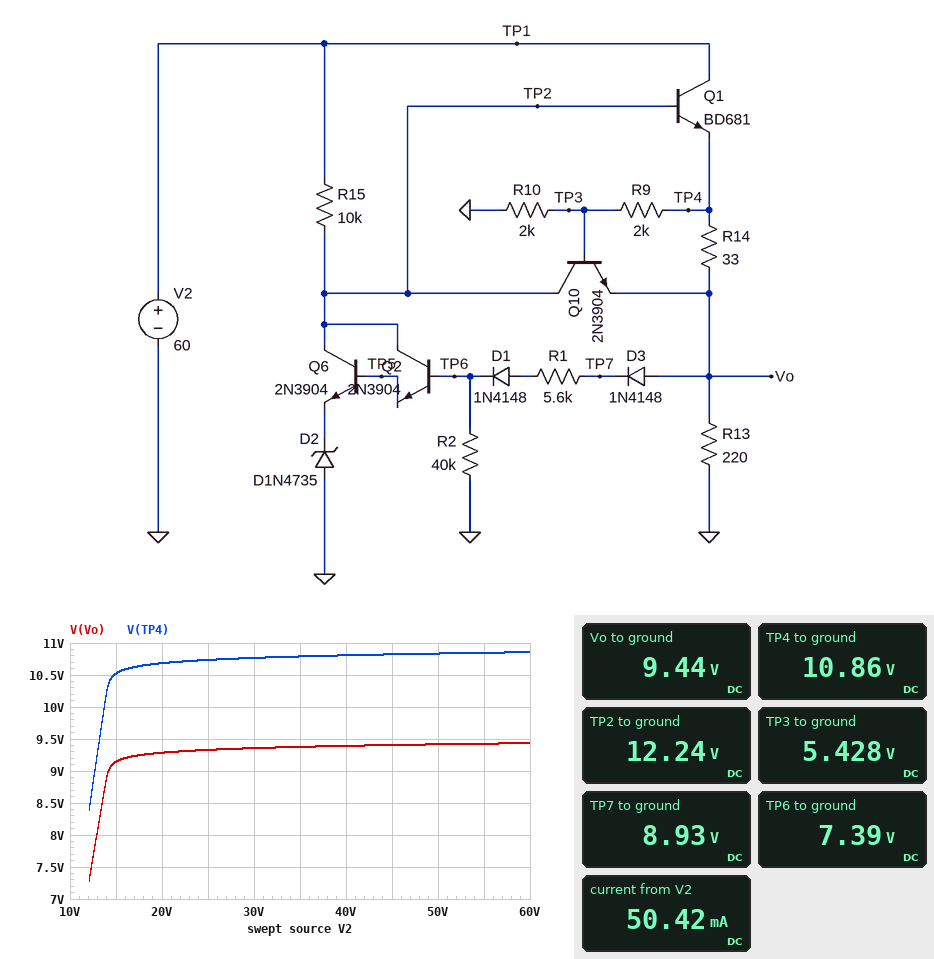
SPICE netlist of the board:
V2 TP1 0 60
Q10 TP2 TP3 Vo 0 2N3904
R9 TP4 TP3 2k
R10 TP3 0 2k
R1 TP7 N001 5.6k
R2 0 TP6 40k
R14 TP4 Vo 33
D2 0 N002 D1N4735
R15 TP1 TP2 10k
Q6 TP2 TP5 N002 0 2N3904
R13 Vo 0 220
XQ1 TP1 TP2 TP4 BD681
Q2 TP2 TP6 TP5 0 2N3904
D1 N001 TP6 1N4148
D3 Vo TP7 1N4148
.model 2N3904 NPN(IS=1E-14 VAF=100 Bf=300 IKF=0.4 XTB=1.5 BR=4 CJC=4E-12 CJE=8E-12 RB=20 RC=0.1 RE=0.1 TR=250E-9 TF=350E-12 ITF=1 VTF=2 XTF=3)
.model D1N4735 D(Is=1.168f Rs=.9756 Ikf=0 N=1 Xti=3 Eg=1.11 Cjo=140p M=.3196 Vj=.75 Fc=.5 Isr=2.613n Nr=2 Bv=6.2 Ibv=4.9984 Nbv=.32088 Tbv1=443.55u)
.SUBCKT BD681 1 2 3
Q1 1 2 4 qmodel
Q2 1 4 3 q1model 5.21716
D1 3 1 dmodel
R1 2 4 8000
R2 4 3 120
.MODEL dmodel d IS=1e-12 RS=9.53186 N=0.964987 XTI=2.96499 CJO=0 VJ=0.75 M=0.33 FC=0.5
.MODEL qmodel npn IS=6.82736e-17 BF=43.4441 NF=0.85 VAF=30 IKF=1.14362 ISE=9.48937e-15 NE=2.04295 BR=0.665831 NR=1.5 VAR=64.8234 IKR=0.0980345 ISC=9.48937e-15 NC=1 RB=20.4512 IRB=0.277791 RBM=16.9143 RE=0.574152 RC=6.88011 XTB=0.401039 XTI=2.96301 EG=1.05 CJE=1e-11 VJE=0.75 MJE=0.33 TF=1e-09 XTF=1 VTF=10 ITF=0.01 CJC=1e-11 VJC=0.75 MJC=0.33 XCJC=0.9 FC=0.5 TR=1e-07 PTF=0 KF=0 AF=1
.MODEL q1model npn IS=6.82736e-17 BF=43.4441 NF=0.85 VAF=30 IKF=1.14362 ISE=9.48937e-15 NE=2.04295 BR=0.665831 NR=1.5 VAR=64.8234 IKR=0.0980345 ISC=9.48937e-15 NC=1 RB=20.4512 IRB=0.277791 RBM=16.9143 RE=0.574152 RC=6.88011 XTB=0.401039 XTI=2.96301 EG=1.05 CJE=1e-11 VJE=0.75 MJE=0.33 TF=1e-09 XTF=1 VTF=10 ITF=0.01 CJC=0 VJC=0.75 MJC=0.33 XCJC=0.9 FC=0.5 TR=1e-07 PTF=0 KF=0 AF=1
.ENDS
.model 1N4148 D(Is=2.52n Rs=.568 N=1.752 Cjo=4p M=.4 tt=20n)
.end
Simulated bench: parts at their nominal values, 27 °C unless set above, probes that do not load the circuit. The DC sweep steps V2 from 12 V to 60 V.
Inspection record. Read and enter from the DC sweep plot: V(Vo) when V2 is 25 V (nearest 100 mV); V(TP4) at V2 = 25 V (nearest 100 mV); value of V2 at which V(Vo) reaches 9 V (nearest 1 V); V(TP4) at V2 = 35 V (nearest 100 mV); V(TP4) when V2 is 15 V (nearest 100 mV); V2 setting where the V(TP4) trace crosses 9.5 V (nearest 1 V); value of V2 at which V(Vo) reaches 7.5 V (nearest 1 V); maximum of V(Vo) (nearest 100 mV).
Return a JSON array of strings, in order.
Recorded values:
["9.3 V", "10.7 V", "14 V", "10.8 V", "10.5 V", "13 V", "12 V", "9.4 V"]
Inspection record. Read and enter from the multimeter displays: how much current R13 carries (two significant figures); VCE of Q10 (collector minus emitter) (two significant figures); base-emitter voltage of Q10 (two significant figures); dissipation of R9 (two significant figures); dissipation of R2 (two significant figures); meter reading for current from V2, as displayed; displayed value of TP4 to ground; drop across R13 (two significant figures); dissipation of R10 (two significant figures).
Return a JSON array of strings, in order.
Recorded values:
["43 mA", "2.8 V", "-4.0 V", "15 mW", "1.4 mW", "50.42 mA", "10.86 V", "9.4 V", "15 mW"]
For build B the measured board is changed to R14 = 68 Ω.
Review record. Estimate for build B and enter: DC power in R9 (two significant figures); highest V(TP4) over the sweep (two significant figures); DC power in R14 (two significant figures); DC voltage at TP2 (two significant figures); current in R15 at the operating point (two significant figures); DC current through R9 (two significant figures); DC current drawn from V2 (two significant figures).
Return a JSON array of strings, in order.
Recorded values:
["19 mW", "12 V", "130 mW", "14 V", "4.6 mA", "3.1 mA", "51 mA"]
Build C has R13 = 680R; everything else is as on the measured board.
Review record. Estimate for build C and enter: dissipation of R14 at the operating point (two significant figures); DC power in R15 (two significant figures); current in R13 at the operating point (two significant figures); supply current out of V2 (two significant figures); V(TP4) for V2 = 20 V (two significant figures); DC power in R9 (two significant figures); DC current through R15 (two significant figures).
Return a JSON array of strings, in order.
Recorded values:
["6.5 mW", "240 mW", "14 mA", "21 mA", "9.8 V", "12 mW", "4.9 mA"]
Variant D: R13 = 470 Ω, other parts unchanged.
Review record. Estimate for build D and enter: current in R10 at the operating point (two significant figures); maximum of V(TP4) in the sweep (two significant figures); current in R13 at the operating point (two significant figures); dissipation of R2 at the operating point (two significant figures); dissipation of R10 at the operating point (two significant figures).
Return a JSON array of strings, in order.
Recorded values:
["2.5 mA", "10 V", "20 mA", "1.4 mW", "13 mW"]
